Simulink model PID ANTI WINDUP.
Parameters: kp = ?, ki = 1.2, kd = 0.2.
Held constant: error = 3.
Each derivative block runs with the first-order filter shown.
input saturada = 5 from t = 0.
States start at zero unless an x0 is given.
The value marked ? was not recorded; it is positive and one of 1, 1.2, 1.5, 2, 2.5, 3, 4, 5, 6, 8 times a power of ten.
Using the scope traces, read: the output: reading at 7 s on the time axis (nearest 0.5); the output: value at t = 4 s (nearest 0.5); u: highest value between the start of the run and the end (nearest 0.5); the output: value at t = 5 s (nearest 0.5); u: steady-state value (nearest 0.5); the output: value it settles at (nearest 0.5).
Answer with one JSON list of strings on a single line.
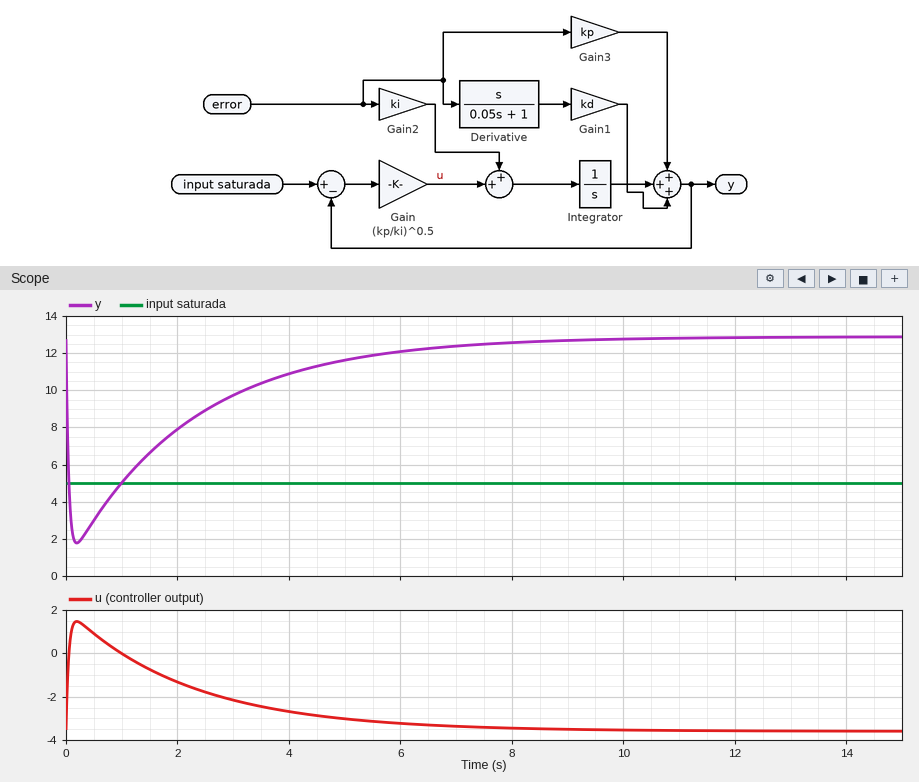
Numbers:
["12.5", "11.0", "1.5", "11.5", "-3.5", "13.0"]
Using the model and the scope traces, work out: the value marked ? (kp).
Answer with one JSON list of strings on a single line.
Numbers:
["0.25"]
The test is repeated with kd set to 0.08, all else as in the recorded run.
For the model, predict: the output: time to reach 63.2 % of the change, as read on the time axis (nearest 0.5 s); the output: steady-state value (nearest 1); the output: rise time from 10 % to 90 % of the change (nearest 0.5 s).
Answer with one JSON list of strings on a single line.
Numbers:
["3.5 s", "13", "5.0 s"]
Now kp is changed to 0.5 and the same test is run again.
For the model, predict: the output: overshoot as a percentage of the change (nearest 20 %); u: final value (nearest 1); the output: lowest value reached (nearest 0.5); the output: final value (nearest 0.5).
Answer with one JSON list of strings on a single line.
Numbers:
["280 %", "-4", "2.5", "10.5"]
